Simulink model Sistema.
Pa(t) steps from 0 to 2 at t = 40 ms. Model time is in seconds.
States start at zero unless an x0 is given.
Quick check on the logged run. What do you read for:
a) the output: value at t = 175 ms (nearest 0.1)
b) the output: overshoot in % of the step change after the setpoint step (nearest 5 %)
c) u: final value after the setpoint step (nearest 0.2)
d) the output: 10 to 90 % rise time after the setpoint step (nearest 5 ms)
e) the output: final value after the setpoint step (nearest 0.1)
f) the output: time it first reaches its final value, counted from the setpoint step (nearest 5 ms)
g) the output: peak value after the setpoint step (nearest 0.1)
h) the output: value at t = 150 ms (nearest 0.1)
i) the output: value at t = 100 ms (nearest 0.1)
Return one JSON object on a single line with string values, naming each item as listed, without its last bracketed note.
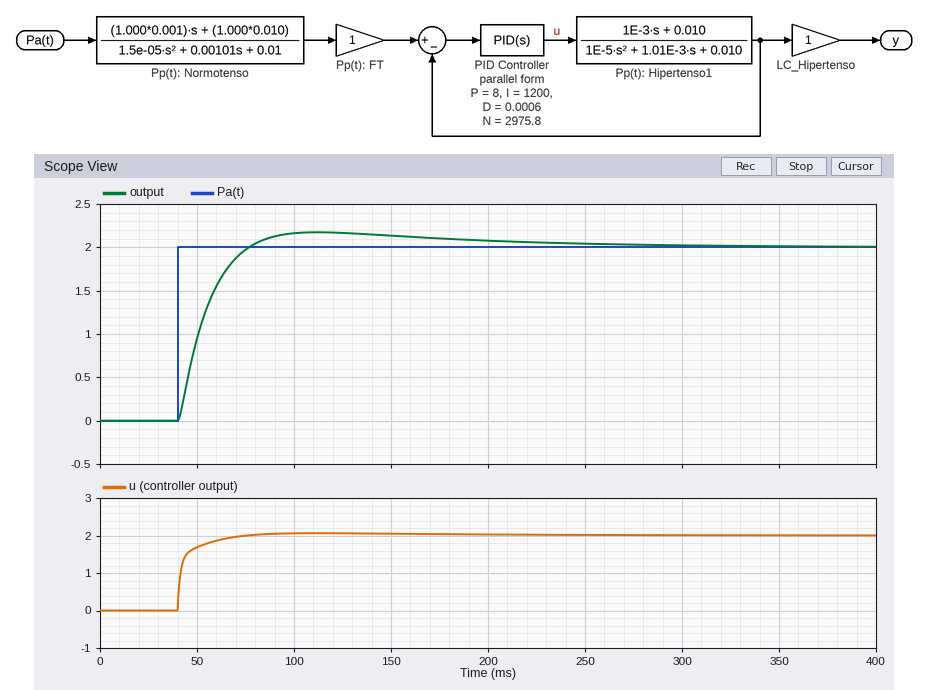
{"the output: value at t = 175 ms": "2.1", "the output: overshoot in % of the step change after the setpoint step": "10 %", "u: final value after the setpoint step": "2.0", "the output: 10 to 90 % rise time after the setpoint step": "25 ms", "the output: final value after the setpoint step": "2.0", "the output: time it first reaches its final value, counted from the setpoint step": "35 ms", "the output: peak value after the setpoint step": "2.2", "the output: value at t = 150 ms": "2.1", "the output: value at t = 100 ms": "2.2"}
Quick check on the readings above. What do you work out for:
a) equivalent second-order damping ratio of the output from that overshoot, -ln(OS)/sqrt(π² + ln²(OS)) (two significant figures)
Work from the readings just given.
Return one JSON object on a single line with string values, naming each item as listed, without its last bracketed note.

{"equivalent second-order damping ratio of the output from that overshoot, -ln(OS)/sqrt(π² + ln²(OS))": "0.59"}
